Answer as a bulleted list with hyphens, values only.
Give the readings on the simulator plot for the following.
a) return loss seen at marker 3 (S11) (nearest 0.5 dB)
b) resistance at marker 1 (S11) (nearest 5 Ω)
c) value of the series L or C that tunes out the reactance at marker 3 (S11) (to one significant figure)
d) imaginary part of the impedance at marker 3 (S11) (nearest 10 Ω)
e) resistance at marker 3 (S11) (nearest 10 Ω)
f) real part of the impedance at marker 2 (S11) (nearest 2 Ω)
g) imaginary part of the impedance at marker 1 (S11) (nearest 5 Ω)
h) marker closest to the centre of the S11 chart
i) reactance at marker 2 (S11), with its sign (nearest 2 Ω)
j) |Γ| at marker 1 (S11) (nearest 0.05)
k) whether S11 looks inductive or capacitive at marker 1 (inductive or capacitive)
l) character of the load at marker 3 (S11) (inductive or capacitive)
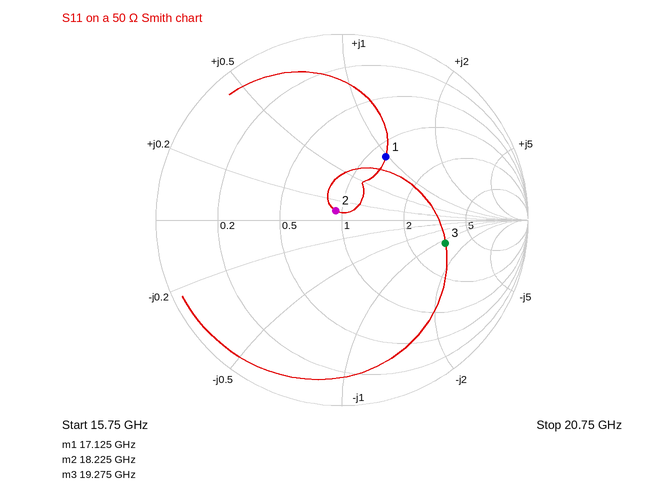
- 5.0 dB
- 60 Ω
- 500 pH
- -60 Ω
- 160 Ω
- 46 Ω
- +50 Ω
- marker 2
- +4 Ω
- 0.40
- inductive
- capacitive
